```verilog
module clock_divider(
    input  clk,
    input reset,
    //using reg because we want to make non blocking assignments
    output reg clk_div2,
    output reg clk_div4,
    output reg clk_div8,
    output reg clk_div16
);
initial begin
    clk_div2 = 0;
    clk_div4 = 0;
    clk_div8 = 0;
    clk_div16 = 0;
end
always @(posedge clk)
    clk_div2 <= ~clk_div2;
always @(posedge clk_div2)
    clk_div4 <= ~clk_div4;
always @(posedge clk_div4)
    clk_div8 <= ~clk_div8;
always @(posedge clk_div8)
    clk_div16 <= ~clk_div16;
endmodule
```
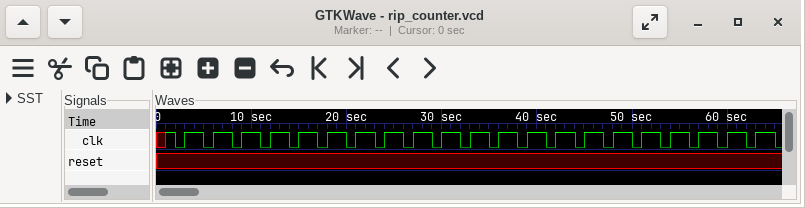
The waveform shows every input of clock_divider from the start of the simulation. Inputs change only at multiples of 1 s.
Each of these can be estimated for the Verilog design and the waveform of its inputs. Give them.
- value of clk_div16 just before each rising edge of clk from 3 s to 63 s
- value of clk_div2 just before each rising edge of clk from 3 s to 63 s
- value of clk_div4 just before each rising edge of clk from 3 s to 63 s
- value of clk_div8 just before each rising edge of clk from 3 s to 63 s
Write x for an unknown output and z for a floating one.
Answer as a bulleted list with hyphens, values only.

- 1 1 1 1 1 1 1 1 0 0 0 0 0 0 0 0 1 1 1 1 1
- 1 0 1 0 1 0 1 0 1 0 1 0 1 0 1 0 1 0 1 0 1
- 1 1 0 0 1 1 0 0 1 1 0 0 1 1 0 0 1 1 0 0 1
- 1 1 1 1 0 0 0 0 1 1 1 1 0 0 0 0 1 1 1 1 0
